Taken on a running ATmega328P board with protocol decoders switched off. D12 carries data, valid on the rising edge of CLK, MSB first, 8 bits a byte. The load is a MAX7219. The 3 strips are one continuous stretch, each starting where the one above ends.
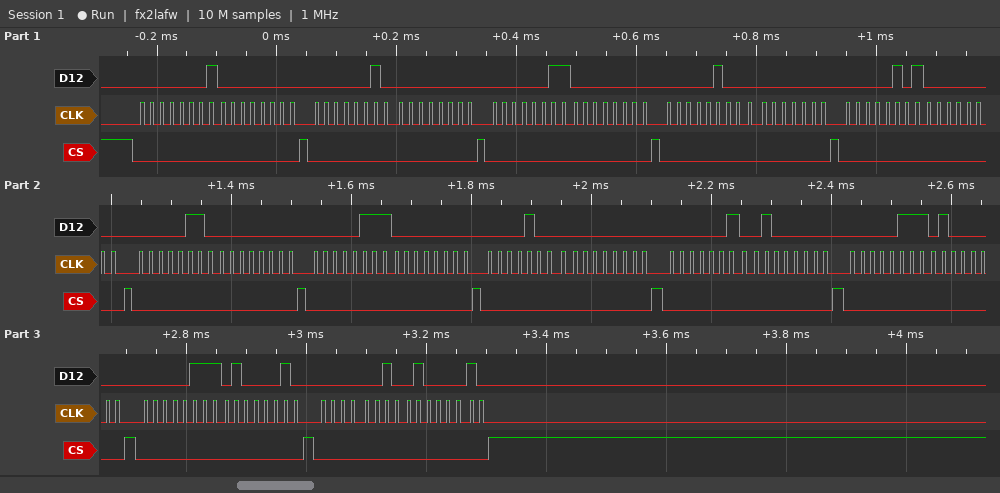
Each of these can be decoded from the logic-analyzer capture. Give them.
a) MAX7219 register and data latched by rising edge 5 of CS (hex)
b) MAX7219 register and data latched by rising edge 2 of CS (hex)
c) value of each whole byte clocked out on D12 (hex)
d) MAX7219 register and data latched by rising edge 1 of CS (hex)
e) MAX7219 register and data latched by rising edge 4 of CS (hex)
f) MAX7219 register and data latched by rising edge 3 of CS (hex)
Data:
register 0x5, data 0x00
register 0x2, data 0x00
01 00 02 00 03 00 04 00 05 00 06 00 07 00 08 00 02 40 07 40 07 42 02 42
register 0x1, data 0x00
register 0x4, data 0x00
register 0x3, data 0x00
